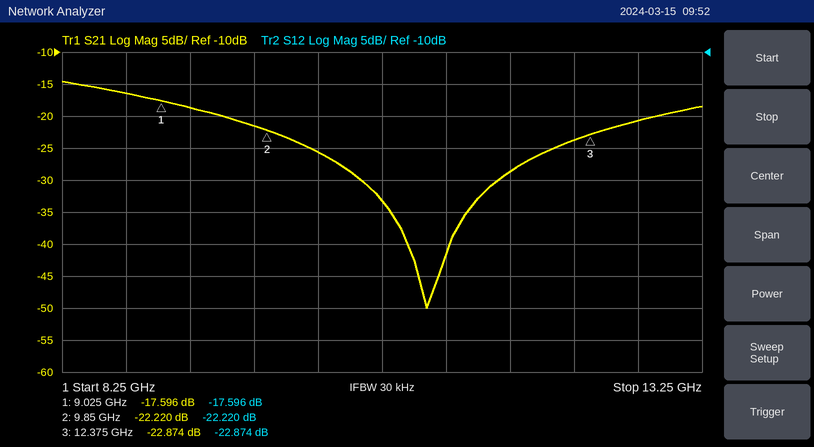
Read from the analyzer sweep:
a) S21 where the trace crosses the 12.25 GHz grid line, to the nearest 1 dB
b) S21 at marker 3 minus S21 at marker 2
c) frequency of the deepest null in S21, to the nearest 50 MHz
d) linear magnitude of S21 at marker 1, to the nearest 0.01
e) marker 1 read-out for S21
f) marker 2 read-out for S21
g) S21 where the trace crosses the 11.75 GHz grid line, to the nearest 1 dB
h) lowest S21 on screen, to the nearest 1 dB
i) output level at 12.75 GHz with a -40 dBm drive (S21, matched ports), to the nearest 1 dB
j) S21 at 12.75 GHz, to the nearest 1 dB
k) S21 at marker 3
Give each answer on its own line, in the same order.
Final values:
-24 dB
-0.654 dB
11.10 GHz
0.13
-17.596 dB
-22.220 dB
-29 dB
-50 dB
-61 dBm
-21 dB
-22.874 dB
